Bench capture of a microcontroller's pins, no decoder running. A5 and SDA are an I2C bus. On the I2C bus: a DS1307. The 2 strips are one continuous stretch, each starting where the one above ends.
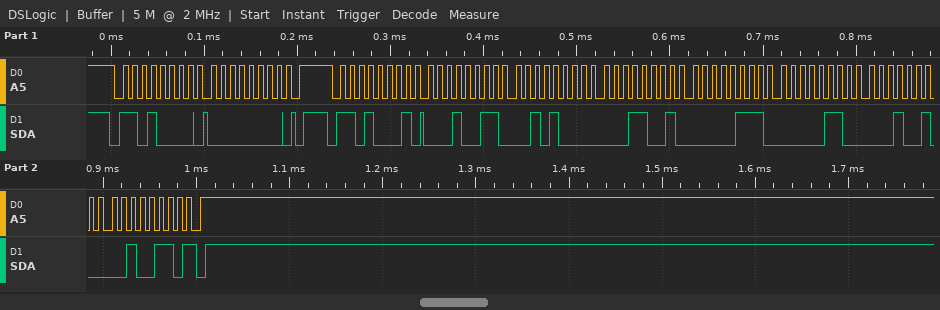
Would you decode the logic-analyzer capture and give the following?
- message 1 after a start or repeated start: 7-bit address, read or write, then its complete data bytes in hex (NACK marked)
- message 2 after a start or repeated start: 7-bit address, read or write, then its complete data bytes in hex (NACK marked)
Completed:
0x68 write: 00
0x68 read: 13 28 19 07 06 12 26 NACK
